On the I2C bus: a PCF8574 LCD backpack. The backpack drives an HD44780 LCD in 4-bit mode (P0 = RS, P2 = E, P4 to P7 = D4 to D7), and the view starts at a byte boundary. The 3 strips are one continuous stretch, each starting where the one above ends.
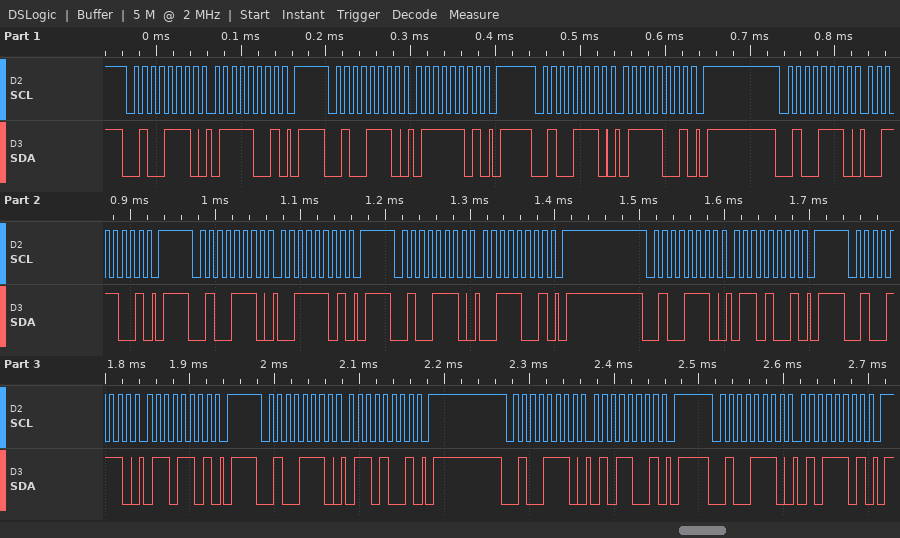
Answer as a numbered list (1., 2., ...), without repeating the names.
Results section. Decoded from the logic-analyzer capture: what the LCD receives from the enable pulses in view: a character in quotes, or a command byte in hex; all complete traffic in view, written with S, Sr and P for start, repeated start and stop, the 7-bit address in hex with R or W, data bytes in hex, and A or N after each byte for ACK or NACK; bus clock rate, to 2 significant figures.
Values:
1. 's'
2. S 27W A 79 A P S 27W A 7D A P S 27W A 79 A P S 27W A 39 A P S 27W A 3D A P S 27W A 39 A P S 27W A 69 A P S 27W A 6D A P S 27W A 69 A P S 27W A 59 A P S 27W A 5D A P
3. 100 kHz
